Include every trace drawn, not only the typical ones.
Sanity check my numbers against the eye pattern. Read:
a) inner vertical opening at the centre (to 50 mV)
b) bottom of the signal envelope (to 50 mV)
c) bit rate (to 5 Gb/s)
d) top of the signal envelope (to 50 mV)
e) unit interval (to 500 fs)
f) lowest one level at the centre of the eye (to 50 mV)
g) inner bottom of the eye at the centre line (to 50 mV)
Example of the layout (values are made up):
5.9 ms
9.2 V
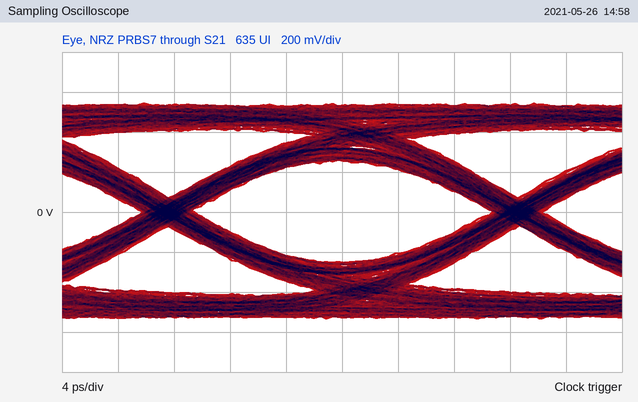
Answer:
500 mV
-550 mV
40 Gb/s
550 mV
25.0 ps
250 mV
-250 mV
